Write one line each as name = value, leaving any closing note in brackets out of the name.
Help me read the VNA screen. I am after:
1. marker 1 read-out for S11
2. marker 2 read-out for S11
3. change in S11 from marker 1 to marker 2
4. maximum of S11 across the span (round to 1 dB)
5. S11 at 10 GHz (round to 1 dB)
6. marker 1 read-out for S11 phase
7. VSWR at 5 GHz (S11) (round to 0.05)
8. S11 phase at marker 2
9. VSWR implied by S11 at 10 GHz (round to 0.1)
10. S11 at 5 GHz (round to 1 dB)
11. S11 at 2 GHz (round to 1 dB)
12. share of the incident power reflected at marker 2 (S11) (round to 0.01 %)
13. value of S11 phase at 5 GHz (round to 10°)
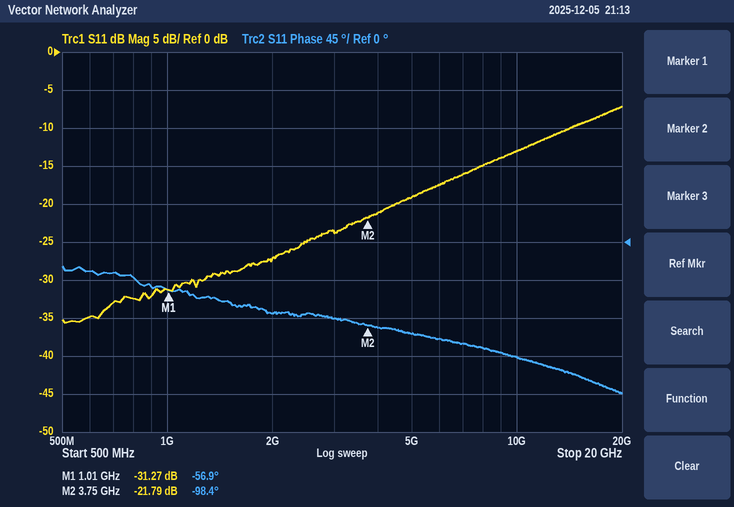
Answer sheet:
marker 1 read-out for S11 = -31.27 dB
marker 2 read-out for S11 = -21.79 dB
change in S11 from marker 1 to marker 2 = 9.48 dB
maximum of S11 across the span = -7 dB
S11 at 10 GHz = -13 dB
marker 1 read-out for S11 phase = -56.9°
VSWR at 5 GHz (S11) = 1.25
S11 phase at marker 2 = -98.4°
VSWR implied by S11 at 10 GHz = 1.6
S11 at 5 GHz = -19 dB
S11 at 2 GHz = -27 dB
share of the incident power reflected at marker 2 (S11) = 0.66 %
value of S11 phase at 5 GHz = -110°
